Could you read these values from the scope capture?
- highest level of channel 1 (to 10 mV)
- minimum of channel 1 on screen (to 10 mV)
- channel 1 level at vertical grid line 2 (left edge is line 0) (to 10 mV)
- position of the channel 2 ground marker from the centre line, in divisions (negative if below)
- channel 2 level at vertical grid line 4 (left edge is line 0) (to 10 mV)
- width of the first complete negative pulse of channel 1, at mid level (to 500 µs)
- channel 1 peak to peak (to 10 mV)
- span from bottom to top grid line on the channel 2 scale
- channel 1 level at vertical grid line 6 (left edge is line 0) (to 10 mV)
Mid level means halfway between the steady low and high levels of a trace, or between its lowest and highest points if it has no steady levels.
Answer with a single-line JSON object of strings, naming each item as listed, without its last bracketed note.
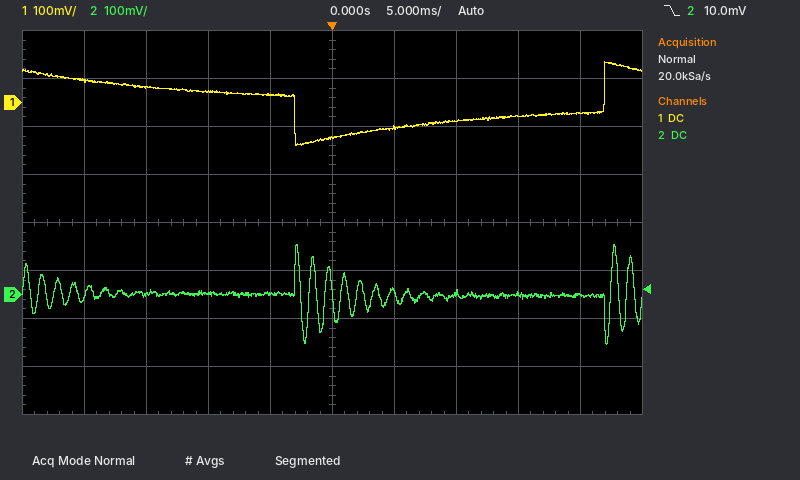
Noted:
{"highest level of channel 1": "90 mV", "minimum of channel 1 on screen": "-90 mV", "channel 1 level at vertical grid line 2 (left edge is line 0)": "30 mV", "position of the channel 2 ground marker from the centre line, in divisions": "-1.5 div", "channel 2 level at vertical grid line 4 (left edge is line 0)": "0 mV", "width of the first complete negative pulse of channel 1, at mid level": "25.0 ms", "channel 1 peak to peak": "180 mV", "span from bottom to top grid line on the channel 2 scale": "800 mV", "channel 1 level at vertical grid line 6 (left edge is line 0)": "-50 mV"}
